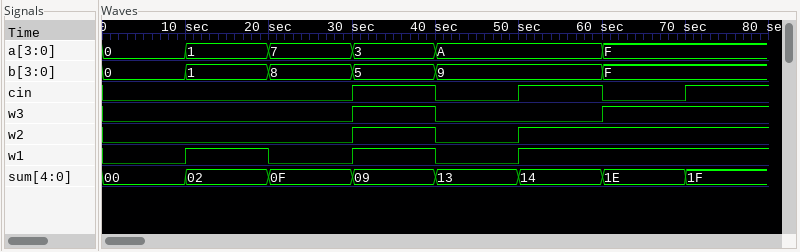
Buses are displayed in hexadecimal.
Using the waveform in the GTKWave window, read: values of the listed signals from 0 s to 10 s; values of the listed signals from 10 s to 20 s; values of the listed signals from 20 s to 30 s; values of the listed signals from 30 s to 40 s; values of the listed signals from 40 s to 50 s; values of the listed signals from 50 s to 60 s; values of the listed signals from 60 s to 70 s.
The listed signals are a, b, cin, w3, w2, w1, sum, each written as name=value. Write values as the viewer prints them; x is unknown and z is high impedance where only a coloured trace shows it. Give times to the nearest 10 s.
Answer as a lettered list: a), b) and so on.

a) a=0, b=0, cin=0, w3=0, w2=0, w1=0, sum=00
b) a=1, b=1, cin=0, w3=0, w2=0, w1=1, sum=02
c) a=7, b=8, cin=0, w3=0, w2=0, w1=0, sum=0F
d) a=3, b=5, cin=1, w3=1, w2=1, w1=1, sum=09
e) a=A, b=9, cin=0, w3=0, w2=0, w1=0, sum=13
f) a=A, b=9, cin=1, w3=0, w2=1, w1=1, sum=14
g) a=F, b=F, cin=0, w3=1, w2=1, w1=1, sum=1E
